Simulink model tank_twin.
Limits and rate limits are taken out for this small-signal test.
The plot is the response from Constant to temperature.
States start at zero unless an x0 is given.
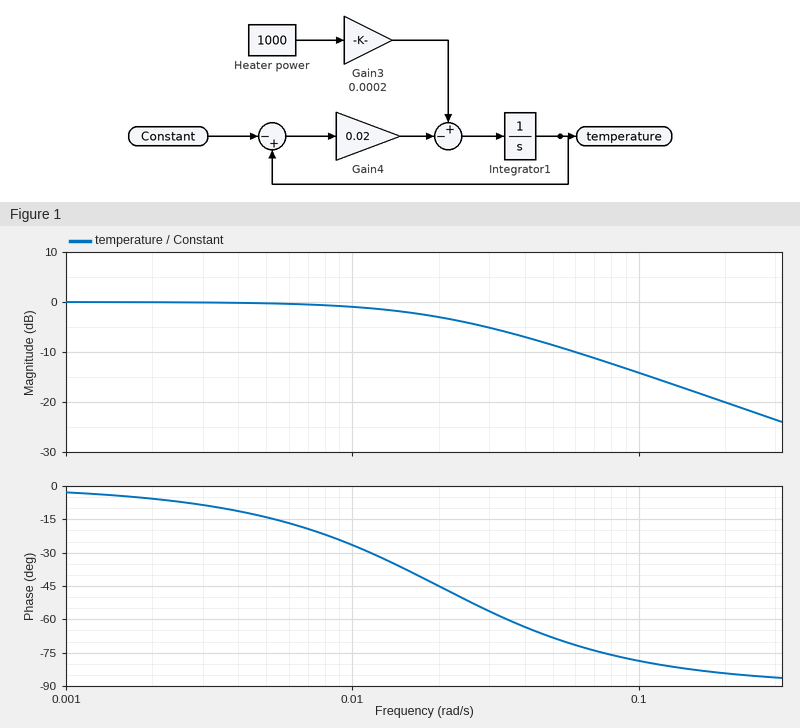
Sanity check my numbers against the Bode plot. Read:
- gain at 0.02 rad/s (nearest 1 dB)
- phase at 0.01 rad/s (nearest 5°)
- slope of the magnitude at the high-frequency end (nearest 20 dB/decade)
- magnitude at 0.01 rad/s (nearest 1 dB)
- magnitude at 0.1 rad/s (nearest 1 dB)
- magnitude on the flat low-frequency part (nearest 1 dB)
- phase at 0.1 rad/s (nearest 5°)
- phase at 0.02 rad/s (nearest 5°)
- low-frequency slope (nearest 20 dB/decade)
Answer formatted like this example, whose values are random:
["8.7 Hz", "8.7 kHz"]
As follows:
["-3 dB", "-25°", "-20 dB/decade", "-1 dB", "-14 dB", "0 dB", "-80°", "-45°", "0 dB/decade"]
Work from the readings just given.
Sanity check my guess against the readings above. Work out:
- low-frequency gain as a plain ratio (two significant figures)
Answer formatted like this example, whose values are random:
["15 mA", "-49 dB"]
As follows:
["1.0"]
